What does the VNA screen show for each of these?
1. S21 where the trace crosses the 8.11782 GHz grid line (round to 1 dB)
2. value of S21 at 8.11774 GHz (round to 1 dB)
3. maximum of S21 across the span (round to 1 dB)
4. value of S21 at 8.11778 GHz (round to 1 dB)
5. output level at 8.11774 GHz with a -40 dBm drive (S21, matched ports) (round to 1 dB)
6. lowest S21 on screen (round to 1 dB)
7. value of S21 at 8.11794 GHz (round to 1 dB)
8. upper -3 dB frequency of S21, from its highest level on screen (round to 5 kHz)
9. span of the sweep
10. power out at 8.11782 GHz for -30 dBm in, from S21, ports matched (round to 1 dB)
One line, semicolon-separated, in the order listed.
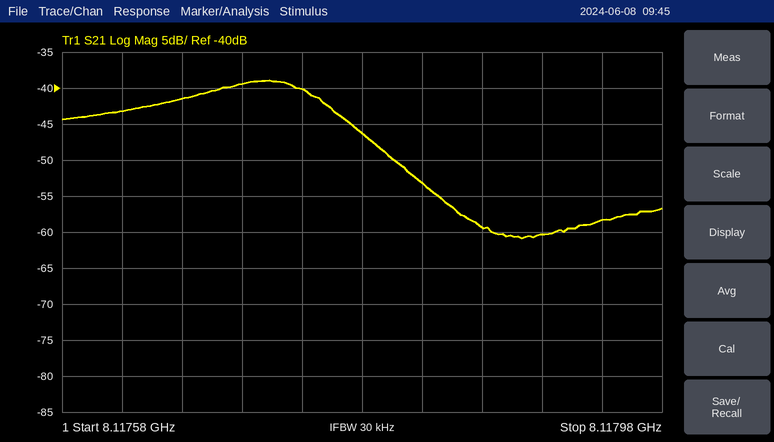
-53 dB; -40 dB; -39 dB; -46 dB; -80 dBm; -61 dB; -58 dB; 8.117755 GHz; 400 kHz; -83 dBm
